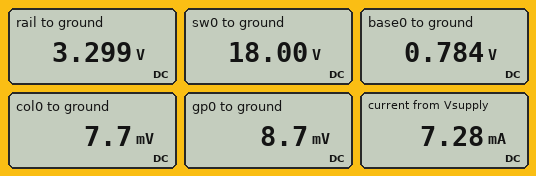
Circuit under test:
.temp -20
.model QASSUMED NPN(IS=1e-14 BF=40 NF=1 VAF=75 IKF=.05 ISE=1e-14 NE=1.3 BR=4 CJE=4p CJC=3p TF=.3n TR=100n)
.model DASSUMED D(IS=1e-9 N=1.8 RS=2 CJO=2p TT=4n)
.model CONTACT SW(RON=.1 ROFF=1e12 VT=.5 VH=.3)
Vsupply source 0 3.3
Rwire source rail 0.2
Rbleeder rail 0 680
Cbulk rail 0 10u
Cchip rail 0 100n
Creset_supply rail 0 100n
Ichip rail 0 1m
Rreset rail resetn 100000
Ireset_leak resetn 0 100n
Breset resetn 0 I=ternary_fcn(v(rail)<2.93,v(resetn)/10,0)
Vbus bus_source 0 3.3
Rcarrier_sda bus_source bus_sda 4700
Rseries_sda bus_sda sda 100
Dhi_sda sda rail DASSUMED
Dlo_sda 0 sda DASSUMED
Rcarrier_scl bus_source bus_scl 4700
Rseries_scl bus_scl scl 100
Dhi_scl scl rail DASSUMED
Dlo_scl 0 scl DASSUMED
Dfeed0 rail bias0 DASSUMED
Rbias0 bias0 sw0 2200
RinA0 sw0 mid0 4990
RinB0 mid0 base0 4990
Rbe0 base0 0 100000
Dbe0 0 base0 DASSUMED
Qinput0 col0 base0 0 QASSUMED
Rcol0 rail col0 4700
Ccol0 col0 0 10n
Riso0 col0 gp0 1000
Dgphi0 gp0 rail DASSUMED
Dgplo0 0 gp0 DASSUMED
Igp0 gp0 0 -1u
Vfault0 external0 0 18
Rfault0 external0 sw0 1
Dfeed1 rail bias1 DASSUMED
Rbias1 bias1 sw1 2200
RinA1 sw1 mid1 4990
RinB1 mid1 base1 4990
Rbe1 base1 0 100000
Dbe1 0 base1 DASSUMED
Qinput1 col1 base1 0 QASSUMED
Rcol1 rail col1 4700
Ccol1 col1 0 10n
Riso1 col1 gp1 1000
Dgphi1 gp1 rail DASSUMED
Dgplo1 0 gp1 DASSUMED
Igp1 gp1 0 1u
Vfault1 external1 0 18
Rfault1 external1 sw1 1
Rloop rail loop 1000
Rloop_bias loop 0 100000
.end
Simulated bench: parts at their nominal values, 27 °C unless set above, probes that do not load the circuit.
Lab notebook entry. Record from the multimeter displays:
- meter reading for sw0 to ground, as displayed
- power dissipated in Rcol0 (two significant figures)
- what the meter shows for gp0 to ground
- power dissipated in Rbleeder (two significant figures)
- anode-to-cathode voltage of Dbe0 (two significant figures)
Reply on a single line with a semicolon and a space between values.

18.00 V; 2.3 mW; 8.7 mV; 16 mW; -780 mV
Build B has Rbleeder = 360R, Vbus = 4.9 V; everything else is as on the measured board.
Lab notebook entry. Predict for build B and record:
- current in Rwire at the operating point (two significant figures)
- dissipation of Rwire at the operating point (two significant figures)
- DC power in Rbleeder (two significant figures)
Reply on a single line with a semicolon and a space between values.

11 mA; 25 µW; 30 mW
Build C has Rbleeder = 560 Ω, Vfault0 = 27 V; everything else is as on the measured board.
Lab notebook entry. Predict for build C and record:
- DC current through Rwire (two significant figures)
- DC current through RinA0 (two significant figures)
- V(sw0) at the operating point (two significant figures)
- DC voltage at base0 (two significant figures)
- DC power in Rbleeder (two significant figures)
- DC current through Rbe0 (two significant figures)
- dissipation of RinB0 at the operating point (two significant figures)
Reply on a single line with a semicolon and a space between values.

8.3 mA; 2.6 mA; 27 V; 790 mV; 19 mW; 7.9 µA; 34 mW
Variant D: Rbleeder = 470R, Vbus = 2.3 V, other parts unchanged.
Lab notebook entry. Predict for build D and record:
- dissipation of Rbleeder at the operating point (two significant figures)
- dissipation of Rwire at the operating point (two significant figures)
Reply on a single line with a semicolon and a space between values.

23 mW; 18 µW
